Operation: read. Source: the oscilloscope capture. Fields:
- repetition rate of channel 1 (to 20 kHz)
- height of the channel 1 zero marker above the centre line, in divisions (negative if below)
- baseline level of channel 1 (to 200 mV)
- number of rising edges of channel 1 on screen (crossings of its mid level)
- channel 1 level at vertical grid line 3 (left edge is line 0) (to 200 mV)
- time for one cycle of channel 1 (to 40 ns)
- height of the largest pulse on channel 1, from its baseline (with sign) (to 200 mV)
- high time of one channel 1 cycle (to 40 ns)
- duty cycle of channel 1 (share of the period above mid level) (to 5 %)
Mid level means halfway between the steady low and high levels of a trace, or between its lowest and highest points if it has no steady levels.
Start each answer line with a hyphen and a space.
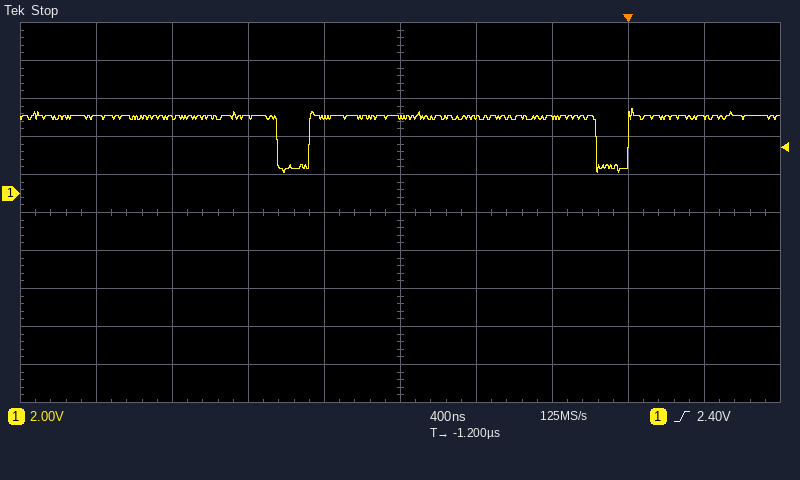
- 600 kHz
- +0.5 div
- 4.0 V
- 2
- 4.0 V
- 1.68 µs
- -3.0 V
- 1.52 µs
- 90 %
